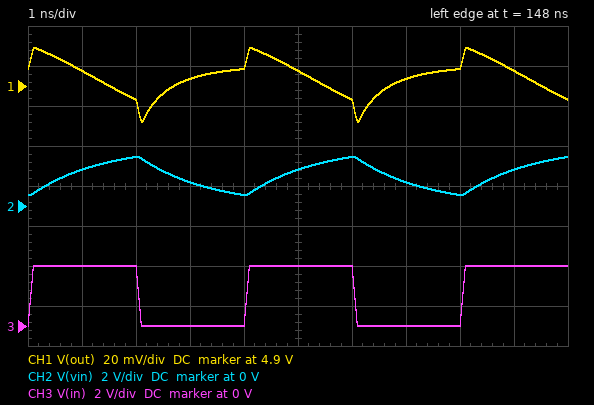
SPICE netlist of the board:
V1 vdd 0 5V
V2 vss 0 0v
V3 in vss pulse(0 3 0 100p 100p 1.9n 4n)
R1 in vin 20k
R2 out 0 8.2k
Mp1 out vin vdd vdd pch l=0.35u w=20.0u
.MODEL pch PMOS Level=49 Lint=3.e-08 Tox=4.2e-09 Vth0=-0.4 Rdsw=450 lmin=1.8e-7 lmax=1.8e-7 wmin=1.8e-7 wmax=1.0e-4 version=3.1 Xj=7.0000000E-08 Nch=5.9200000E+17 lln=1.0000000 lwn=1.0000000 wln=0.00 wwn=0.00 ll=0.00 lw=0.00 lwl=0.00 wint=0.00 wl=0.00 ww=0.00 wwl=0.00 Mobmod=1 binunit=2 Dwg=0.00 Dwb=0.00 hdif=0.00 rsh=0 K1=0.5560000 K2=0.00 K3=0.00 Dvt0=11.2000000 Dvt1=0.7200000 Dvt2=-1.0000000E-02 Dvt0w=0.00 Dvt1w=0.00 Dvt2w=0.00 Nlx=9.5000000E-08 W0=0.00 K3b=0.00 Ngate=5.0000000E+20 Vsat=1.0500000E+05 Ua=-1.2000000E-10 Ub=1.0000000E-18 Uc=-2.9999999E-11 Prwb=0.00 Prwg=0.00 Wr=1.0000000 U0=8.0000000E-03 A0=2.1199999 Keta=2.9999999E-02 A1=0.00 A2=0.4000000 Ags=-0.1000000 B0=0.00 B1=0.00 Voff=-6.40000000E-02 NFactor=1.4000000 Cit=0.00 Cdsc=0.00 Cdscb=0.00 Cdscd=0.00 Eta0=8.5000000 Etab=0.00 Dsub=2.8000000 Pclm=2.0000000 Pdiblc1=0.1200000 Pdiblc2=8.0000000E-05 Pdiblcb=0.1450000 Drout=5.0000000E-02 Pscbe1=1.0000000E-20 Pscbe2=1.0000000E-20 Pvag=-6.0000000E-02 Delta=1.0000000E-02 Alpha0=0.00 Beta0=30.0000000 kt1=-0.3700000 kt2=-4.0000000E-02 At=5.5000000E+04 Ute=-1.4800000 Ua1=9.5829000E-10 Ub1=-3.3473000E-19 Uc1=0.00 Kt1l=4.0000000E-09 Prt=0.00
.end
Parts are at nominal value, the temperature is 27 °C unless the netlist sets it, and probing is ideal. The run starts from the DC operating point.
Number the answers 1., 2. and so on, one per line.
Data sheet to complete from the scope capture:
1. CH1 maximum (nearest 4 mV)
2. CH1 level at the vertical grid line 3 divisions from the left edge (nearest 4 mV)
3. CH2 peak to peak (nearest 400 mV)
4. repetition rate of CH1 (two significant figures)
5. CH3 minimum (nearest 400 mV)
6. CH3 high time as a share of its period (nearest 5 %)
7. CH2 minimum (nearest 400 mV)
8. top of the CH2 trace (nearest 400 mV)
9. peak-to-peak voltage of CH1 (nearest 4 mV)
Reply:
1. 4.920 V
2. 4.904 V
3. 2.0 V
4. 250 MHz
5. 0 V
6. 50 %
7. 400 mV
8. 2.4 V
9. 36 mV
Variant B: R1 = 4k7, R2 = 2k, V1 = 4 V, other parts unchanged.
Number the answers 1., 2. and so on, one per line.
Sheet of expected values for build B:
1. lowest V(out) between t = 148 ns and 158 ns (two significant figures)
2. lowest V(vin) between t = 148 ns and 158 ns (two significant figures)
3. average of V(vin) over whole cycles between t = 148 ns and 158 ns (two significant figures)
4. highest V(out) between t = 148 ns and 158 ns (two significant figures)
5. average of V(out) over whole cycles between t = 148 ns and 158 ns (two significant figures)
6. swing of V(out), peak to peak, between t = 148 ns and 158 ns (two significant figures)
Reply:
1. 1.5 V
2. 5.8 mV
3. 1.5 V
4. 3.7 V
5. 3.0 V
6. 2.3 V
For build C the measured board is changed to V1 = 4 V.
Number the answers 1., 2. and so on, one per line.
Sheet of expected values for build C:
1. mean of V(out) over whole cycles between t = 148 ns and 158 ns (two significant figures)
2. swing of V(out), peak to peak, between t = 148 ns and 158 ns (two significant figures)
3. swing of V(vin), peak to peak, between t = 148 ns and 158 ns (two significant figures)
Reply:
1. 3.9 V
2. 79 mV
3. 1.9 V
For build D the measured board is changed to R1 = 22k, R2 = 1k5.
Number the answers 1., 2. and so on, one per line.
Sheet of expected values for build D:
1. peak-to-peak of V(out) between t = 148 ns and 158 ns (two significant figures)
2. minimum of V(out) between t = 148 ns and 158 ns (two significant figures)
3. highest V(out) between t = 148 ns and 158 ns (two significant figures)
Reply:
1. 180 mV
2. 4.3 V
3. 4.5 V
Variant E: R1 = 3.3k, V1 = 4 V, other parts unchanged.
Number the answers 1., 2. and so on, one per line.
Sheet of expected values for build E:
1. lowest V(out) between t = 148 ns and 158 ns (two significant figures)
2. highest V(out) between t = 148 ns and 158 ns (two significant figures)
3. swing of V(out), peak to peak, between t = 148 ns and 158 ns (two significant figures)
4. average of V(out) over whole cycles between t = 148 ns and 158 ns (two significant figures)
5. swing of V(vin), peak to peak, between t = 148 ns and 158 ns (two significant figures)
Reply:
1. 3.5 V
2. 4.0 V
3. 450 mV
4. 3.8 V
5. 3.0 V
